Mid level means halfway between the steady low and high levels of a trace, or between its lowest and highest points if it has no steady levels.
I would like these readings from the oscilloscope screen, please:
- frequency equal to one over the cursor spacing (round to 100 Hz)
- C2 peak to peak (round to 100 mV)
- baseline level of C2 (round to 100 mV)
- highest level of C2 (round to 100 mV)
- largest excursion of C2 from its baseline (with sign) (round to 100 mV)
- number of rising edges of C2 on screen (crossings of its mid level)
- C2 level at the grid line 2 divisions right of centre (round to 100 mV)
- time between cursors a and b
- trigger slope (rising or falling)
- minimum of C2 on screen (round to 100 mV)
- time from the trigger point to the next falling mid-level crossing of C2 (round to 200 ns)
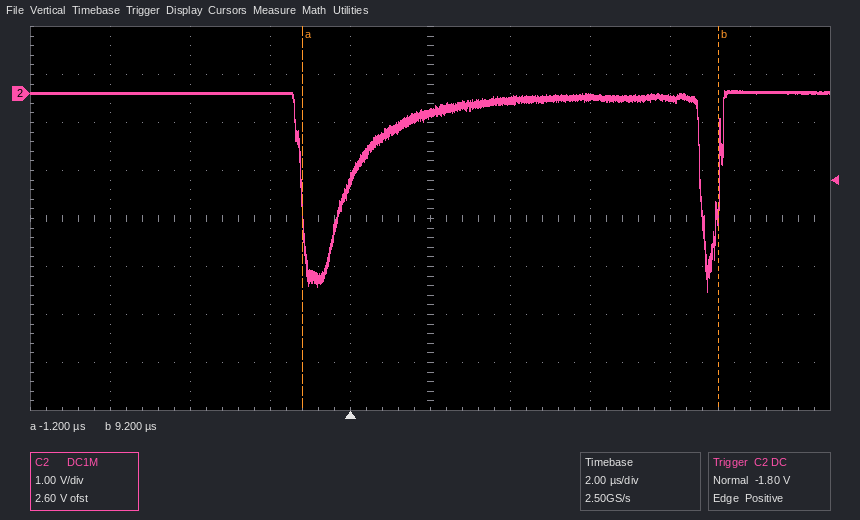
96.2 kHz
4.2 V
0.0 V
100 mV
-4.1 V
2
-100 mV
10.4 µs
rising
-4.1 V
8.8 µs
